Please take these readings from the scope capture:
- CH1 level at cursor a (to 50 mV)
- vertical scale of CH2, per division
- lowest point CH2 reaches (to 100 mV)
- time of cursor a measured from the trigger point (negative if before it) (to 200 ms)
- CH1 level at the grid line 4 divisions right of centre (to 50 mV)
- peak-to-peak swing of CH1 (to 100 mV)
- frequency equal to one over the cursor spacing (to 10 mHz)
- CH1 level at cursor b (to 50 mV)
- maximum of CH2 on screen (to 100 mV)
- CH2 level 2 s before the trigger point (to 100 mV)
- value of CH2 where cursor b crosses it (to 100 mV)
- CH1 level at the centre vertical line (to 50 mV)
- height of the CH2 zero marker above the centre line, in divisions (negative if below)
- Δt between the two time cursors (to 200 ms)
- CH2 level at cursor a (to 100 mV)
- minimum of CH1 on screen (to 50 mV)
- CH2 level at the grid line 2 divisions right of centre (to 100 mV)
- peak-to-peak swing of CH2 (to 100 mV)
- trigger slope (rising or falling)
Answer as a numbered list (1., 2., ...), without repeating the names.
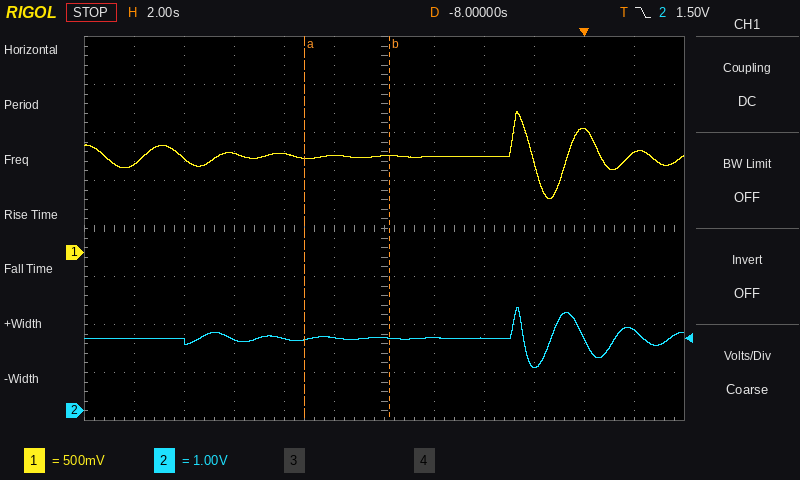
1. 1.00 V
2. 1 V
3. 900 mV
4. -11.2 s
5. 1.30 V
6. 900 mV
7. 290 mHz
8. 1.00 V
9. 2.2 V
10. 900 mV
11. 1.5 V
12. 1.00 V
13. -3.8 div
14. 3.4 s
15. 1.5 V
16. 550 mV
17. 1.5 V
18. 1.3 V
19. falling
